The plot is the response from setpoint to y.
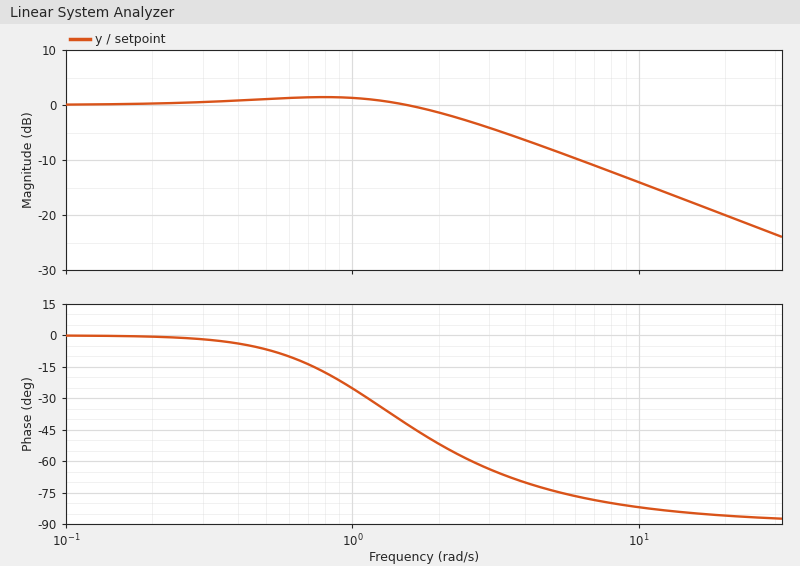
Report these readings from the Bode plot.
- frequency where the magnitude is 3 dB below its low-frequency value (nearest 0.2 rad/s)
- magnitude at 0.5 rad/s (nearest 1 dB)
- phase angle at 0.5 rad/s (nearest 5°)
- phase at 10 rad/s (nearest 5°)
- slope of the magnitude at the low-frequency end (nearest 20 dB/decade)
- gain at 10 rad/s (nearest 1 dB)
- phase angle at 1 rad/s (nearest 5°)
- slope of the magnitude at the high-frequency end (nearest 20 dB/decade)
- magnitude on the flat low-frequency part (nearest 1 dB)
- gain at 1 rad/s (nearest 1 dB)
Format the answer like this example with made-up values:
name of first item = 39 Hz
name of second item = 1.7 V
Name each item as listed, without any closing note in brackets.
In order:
frequency where the magnitude is 3 dB below its low-frequency value = 2.6 rad/s
magnitude at 0.5 rad/s = 1 dB
phase angle at 0.5 rad/s = -5°
phase at 10 rad/s = -80°
slope of the magnitude at the low-frequency end = 0 dB/decade
gain at 10 rad/s = -14 dB
phase angle at 1 rad/s = -25°
slope of the magnitude at the high-frequency end = -20 dB/decade
magnitude on the flat low-frequency part = 0 dB
gain at 1 rad/s = 1 dB
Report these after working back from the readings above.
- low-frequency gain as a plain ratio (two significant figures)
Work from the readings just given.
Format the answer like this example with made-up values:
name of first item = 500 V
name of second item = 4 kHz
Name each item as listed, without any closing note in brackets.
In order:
low-frequency gain as a plain ratio = 1.0
